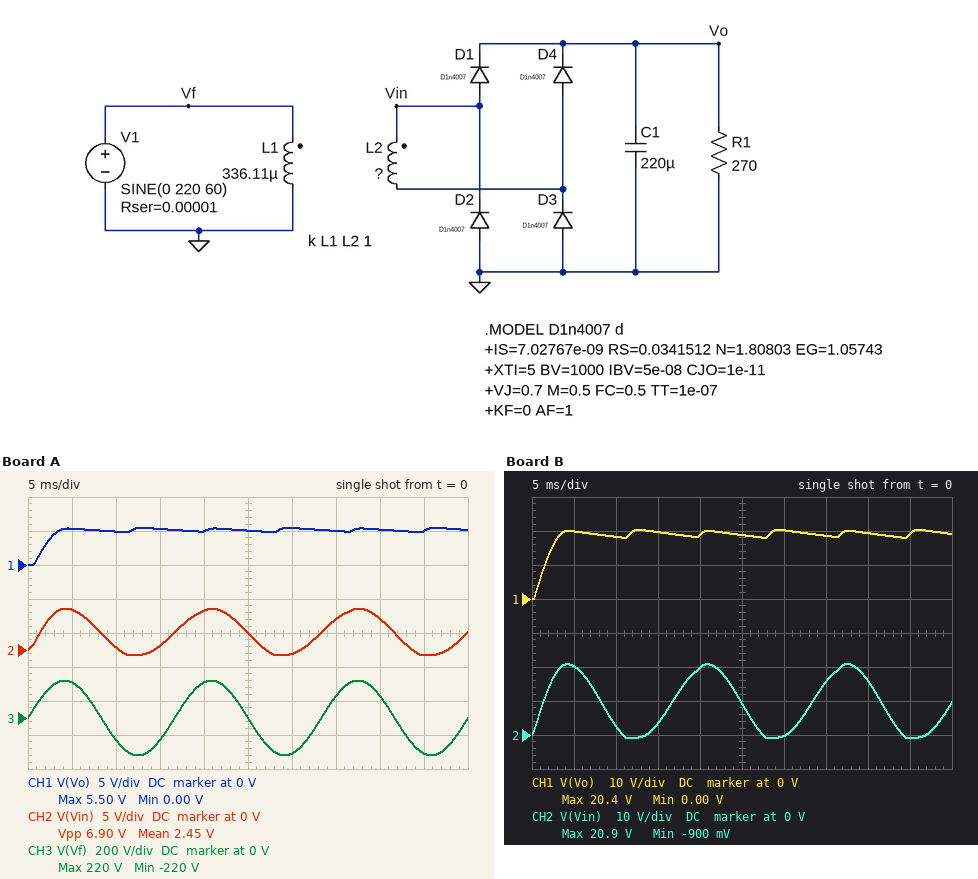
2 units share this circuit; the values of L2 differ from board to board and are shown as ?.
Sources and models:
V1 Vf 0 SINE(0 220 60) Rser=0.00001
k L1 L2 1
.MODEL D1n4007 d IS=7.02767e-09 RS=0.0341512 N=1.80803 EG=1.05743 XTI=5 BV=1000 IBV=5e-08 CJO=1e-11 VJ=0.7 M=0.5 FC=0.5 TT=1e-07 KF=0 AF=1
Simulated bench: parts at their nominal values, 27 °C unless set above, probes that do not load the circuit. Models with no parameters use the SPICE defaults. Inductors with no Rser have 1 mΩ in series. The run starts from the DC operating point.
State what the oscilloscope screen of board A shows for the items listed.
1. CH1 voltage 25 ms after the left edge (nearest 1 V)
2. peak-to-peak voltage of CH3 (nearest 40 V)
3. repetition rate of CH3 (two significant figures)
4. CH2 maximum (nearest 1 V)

5 V
440 V
60 Hz
6 V
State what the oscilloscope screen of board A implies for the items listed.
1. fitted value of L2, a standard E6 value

330 nH
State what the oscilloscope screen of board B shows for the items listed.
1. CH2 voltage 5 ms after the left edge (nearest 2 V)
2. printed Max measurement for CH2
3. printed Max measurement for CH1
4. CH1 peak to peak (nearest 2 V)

20 V
20.9 V
20.4 V
20 V
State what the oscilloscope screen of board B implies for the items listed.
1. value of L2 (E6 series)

3.3 µH
